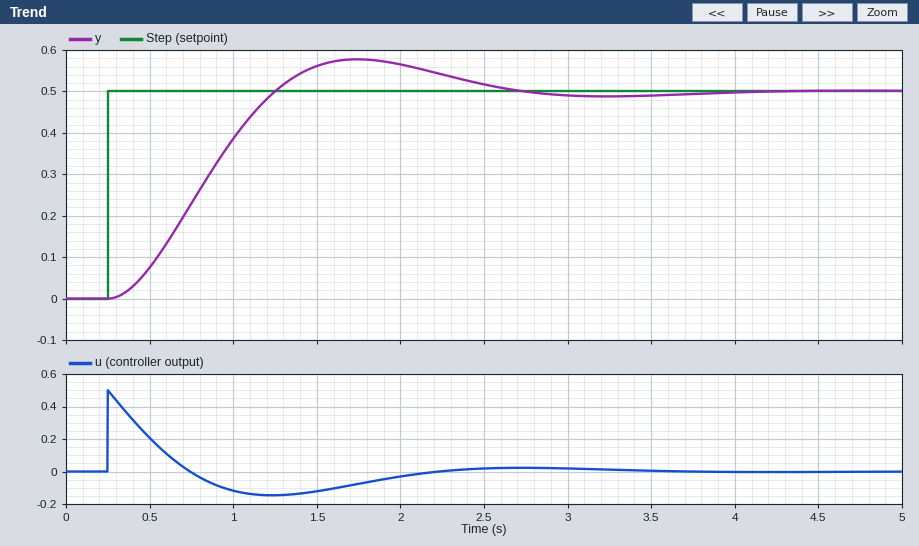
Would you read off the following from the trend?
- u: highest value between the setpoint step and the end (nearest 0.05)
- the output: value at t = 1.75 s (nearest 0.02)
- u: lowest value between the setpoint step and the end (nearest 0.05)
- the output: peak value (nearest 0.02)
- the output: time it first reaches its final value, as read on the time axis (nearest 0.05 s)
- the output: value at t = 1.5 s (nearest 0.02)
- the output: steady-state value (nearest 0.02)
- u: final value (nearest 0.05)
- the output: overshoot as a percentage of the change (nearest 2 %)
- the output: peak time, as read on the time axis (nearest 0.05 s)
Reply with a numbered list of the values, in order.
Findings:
1. 0.50
2. 0.58
3. -0.15
4. 0.58
5. 1.25 s
6. 0.56
7. 0.50
8. 0.00
9. 16 %
10. 1.75 s
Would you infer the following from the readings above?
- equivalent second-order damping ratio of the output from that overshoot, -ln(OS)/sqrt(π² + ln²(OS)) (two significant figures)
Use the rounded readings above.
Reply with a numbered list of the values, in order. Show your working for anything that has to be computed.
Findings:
1. ln(0.16) = -1.833; 1.833 / sqrt(9.870 + 3.358) = 0.50
